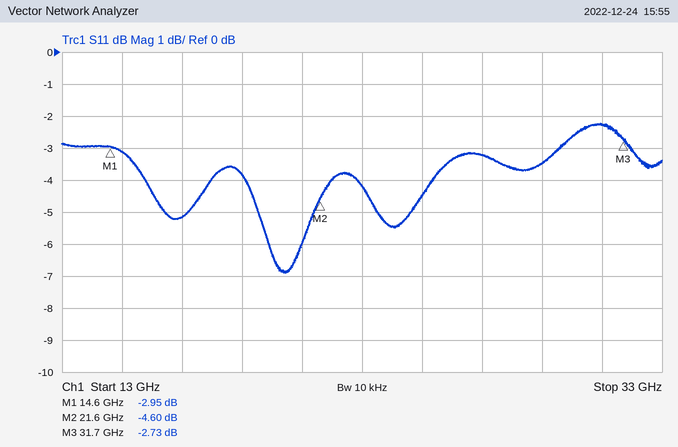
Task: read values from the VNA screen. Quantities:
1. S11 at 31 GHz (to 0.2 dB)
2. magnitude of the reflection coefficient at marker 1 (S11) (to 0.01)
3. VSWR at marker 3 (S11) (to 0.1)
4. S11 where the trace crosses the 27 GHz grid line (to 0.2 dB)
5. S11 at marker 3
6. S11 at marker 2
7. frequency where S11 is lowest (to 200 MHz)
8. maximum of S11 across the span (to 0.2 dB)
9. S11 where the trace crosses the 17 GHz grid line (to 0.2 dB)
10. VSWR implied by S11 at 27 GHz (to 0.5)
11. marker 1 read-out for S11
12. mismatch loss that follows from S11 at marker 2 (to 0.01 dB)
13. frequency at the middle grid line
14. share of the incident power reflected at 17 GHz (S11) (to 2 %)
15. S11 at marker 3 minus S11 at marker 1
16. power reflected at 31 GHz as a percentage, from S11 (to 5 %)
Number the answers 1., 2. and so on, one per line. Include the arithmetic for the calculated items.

1. -2.2 dB
2. 10^(-2.95/20) ≈ 0.71
3. (1 + 0.7303)/(1 − 0.7303) ≈ 6.4
4. -3.2 dB
5. -2.73 dB
6. -4.60 dB
7. 20.4 GHz
8. -2.2 dB
9. -5.2 dB
10. |Γ| = 10^(-3.2/20) = 0.6918; VSWR = (1 + 0.6918)/(1 − 0.6918) ≈ 5.5
11. -2.95 dB
12. −10 log10(1 − 10^(-4.6/10)) ≈ 1.85 dB
13. 23 GHz
14. 10^(-5.2/10) ≈ 30 %
15. -2.73 − (-2.95) = 0.22 dB
16. 10^(-2.2/10) ≈ 60 %
